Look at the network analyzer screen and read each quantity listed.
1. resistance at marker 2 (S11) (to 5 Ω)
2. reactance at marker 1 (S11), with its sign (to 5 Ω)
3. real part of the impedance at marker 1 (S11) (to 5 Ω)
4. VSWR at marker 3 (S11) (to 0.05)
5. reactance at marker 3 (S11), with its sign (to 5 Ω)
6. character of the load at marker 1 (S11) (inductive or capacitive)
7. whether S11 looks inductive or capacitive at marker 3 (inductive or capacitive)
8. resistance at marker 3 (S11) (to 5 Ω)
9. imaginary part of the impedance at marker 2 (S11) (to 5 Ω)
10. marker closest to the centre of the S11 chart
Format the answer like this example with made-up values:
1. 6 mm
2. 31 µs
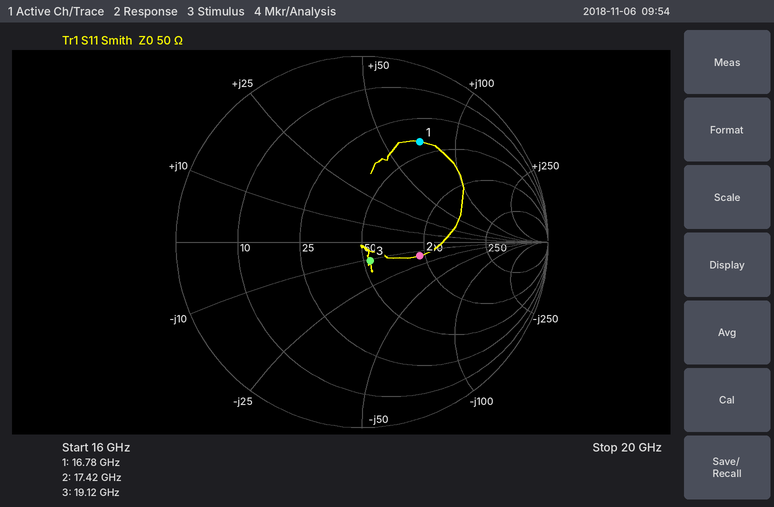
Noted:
1. 95 Ω
2. +70 Ω
3. 40 Ω
4. 1.25
5. -10 Ω
6. inductive
7. capacitive
8. 55 Ω
9. -15 Ω
10. marker 3
